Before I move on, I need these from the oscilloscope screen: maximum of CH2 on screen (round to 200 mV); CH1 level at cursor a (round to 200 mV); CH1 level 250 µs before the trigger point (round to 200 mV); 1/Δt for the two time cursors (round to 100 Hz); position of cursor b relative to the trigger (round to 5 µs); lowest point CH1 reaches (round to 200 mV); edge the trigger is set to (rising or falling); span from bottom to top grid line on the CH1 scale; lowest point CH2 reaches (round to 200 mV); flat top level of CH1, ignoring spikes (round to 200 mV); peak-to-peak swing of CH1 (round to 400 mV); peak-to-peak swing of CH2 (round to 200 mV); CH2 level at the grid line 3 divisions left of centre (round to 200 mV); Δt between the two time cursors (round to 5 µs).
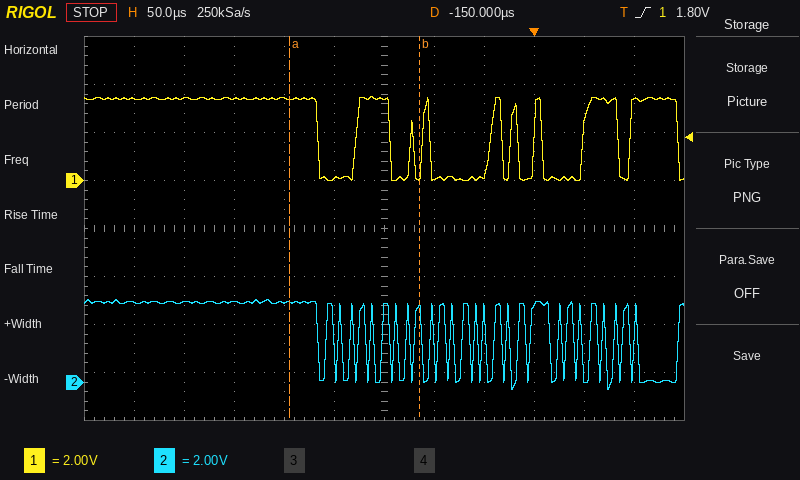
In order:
3.4 V
3.4 V
3.4 V
7.7 kHz
-115 µs
0.0 V
rising
16 V
-400 mV
3.4 V
3.6 V
3.8 V
3.4 V
130 µs
